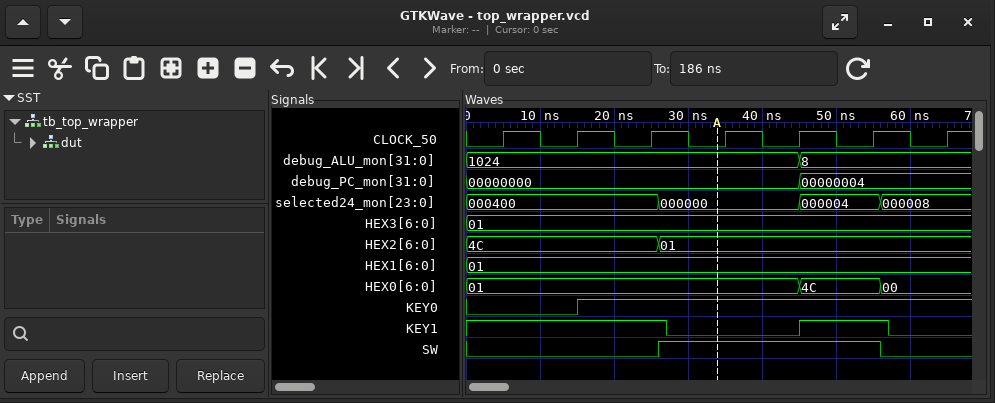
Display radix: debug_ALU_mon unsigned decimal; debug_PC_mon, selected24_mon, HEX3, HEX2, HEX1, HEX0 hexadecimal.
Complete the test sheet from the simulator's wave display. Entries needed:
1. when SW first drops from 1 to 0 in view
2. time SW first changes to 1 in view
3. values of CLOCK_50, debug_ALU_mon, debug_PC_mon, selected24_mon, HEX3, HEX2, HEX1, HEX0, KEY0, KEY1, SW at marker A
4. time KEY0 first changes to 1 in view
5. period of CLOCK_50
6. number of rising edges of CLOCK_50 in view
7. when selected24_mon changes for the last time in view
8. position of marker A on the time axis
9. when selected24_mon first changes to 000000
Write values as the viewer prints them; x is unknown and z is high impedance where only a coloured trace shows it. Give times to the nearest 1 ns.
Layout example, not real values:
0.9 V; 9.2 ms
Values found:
56 ns; 26 ns; CLOCK_50=0, debug_ALU_mon=1024, debug_PC_mon=00000000, selected24_mon=000000, HEX3=01, HEX2=01, HEX1=01, HEX0=01, KEY0=1, KEY1=0, SW=1; 15 ns; 10 ns; 7; 56 ns; 34 ns; 26 ns
